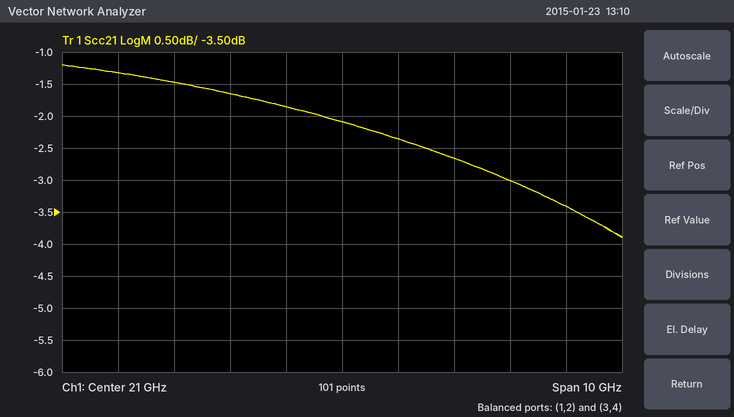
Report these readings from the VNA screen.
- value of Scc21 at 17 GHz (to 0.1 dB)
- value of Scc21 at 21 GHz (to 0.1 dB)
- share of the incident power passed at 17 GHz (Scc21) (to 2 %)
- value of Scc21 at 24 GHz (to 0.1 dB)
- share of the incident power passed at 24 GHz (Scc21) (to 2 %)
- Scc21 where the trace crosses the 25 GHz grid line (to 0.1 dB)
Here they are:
-1.3 dB
-2.1 dB
74 %
-3.0 dB
50 %
-3.4 dB
